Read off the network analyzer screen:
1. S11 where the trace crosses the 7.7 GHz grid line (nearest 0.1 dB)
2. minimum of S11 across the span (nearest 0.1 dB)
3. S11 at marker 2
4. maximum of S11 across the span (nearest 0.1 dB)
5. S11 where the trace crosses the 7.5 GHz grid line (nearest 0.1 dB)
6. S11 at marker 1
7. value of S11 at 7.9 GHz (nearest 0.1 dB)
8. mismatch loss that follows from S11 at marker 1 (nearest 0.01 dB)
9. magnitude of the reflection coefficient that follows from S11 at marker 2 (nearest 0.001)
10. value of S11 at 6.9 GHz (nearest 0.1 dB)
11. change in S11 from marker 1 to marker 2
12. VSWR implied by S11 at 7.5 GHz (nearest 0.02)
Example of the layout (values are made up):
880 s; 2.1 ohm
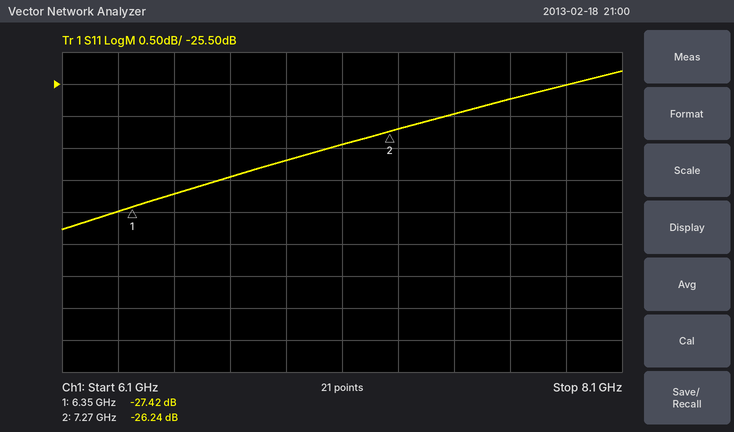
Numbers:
-25.7 dB; -27.8 dB; -26.24 dB; -25.3 dB; -26.0 dB; -27.42 dB; -25.5 dB; 0.01 dB; 0.049; -26.7 dB; 1.18 dB; 1.10
